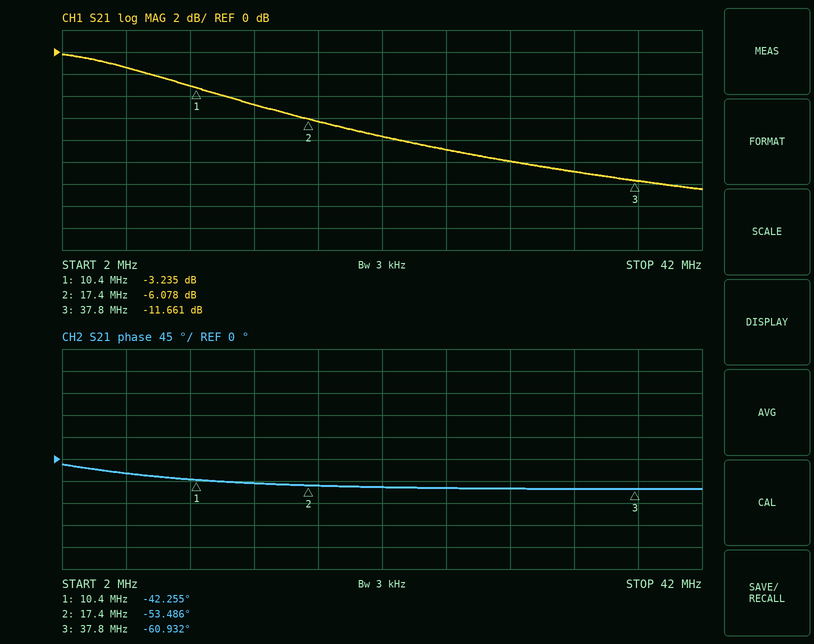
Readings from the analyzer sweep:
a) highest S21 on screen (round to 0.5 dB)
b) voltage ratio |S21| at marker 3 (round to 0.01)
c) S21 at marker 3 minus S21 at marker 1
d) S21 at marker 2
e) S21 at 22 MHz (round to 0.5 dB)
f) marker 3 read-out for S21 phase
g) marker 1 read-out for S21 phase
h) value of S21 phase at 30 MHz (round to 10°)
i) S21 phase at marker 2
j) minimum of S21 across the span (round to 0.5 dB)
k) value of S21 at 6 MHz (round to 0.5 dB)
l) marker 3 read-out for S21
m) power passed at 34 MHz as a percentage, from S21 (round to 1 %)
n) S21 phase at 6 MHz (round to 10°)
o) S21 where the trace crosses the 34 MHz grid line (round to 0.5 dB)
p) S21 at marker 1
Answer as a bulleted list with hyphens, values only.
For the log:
- 0.0 dB
- 0.26
- -8.426 dB
- -6.078 dB
- -7.5 dB
- -60.932°
- -42.255°
- -60°
- -53.486°
- -12.5 dB
- -1.5 dB
- -11.661 dB
- 8 %
- -30°
- -11.0 dB
- -3.235 dB
